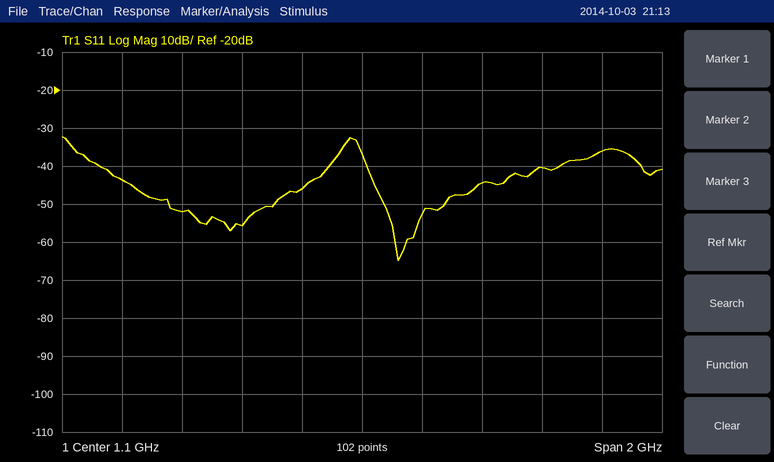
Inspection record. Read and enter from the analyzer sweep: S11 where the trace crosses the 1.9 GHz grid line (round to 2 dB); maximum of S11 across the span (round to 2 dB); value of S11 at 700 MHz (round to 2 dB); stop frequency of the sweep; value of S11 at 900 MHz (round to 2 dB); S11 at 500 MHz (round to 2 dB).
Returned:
-36 dB
-32 dB
-56 dB
2.1 GHz
-46 dB
-52 dB
